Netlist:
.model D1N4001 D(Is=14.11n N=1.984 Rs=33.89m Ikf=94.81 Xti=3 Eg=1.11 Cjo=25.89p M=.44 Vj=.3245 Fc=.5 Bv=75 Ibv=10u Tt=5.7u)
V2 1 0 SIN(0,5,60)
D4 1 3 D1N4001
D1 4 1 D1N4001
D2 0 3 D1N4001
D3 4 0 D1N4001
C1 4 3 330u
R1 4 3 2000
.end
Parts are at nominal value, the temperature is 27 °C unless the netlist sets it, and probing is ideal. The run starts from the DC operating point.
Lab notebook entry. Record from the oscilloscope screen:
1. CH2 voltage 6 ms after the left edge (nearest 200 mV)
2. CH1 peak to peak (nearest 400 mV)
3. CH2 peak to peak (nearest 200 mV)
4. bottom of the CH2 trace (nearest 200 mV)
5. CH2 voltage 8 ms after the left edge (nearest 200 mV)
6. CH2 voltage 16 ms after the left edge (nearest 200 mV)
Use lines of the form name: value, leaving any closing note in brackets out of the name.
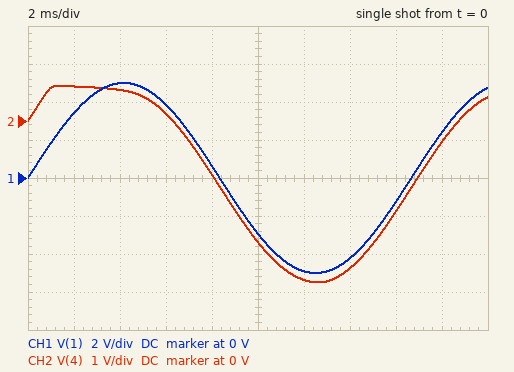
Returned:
CH2 voltage 6 ms after the left edge: 200 mV
CH1 peak to peak: 10.0 V
CH2 peak to peak: 5.2 V
bottom of the CH2 trace: -4.2 V
CH2 voltage 8 ms after the left edge: -1.4 V
CH2 voltage 16 ms after the left edge: -2.4 V
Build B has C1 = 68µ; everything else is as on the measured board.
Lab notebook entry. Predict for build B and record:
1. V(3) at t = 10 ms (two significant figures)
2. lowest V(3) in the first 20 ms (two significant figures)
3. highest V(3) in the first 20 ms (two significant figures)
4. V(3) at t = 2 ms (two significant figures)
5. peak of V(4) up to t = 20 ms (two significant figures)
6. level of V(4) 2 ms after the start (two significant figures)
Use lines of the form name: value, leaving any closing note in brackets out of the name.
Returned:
V(3) at t = 10 ms: 280 mV
lowest V(3) in the first 20 ms: -720 mV
highest V(3) in the first 20 ms: 4.3 V
V(3) at t = 2 ms: 2.6 V
peak of V(4) up to t = 20 ms: 820 mV
level of V(4) 2 ms after the start: 810 mV
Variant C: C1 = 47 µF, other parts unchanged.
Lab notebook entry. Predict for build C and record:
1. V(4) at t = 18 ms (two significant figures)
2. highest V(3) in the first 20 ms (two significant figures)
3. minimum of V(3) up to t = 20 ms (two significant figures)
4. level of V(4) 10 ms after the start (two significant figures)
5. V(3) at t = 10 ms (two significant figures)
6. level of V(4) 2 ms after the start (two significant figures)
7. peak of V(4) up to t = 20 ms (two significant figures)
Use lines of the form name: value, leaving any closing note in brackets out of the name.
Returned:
V(4) at t = 18 ms: -540 mV
highest V(3) in the first 20 ms: 4.3 V
minimum of V(3) up to t = 20 ms: -710 mV
level of V(4) 10 ms after the start: -3.2 V
V(3) at t = 10 ms: 260 mV
level of V(4) 2 ms after the start: 790 mV
peak of V(4) up to t = 20 ms: 800 mV
